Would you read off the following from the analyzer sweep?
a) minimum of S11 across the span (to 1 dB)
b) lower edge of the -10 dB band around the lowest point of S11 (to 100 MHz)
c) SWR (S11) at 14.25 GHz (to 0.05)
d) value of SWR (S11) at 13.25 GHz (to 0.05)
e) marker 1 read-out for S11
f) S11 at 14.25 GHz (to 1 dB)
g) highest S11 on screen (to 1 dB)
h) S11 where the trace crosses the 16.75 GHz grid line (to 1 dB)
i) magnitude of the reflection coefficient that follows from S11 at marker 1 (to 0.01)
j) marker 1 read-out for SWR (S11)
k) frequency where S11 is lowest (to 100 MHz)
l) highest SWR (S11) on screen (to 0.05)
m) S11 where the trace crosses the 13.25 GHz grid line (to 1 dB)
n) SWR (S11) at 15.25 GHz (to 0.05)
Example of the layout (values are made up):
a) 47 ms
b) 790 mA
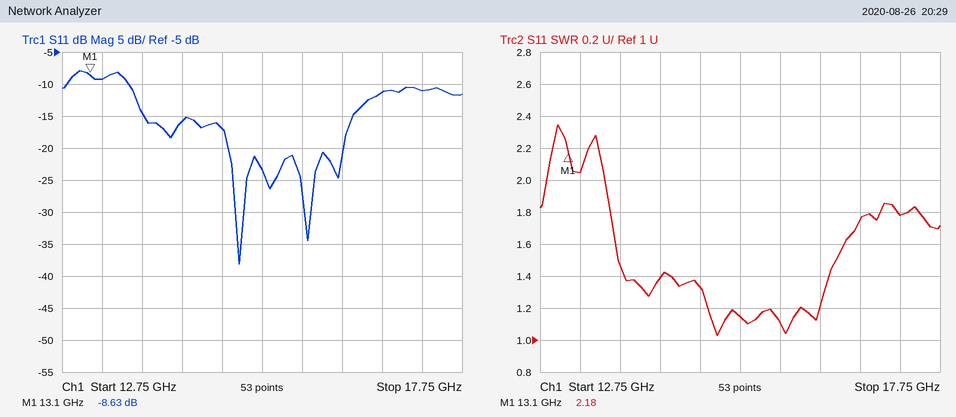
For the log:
a) -38 dB
b) 13.6 GHz
c) 1.40
d) 2.05
e) -8.63 dB
f) -16 dB
g) -8 dB
h) -11 dB
i) 0.37
j) 2.18
k) 15.0 GHz
l) 2.35
m) -9 dB
n) 1.15
